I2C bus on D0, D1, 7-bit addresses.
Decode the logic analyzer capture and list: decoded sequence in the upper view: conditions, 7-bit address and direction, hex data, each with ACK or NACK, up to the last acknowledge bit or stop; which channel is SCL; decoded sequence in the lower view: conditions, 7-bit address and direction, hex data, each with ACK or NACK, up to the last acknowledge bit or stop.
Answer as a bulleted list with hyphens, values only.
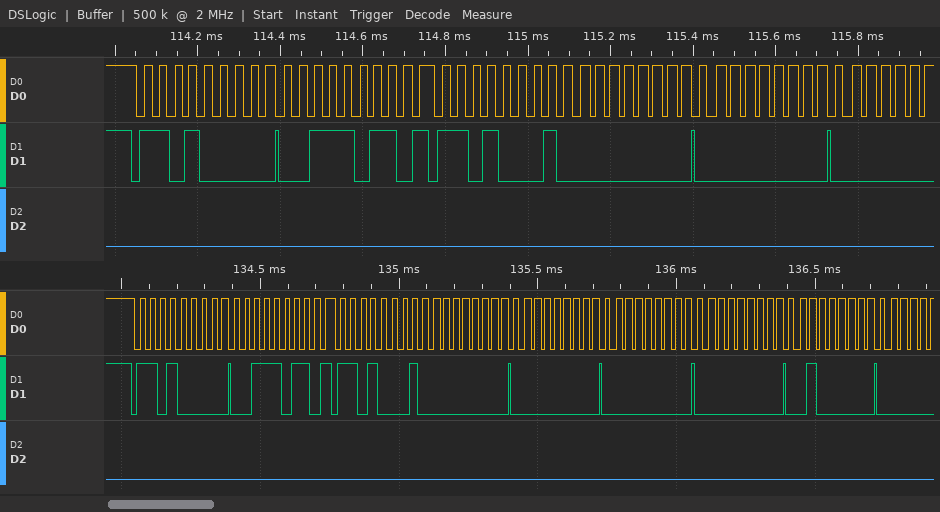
- start, address 68 write ACK, 3B ACK, repeated start, address 68 read ACK, 00 ACK, 00 ACK
- D0
- start, address 68 write ACK, 3B ACK, repeated start, address 68 read ACK, 00 ACK, 00 ACK, 00 ACK, 00 ACK, 40 ACK
